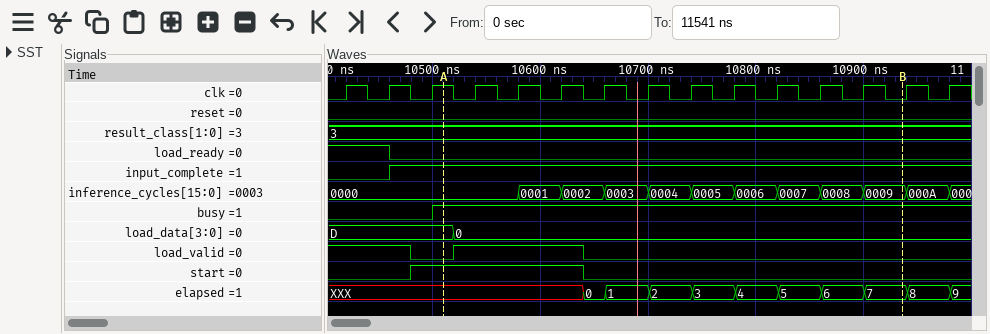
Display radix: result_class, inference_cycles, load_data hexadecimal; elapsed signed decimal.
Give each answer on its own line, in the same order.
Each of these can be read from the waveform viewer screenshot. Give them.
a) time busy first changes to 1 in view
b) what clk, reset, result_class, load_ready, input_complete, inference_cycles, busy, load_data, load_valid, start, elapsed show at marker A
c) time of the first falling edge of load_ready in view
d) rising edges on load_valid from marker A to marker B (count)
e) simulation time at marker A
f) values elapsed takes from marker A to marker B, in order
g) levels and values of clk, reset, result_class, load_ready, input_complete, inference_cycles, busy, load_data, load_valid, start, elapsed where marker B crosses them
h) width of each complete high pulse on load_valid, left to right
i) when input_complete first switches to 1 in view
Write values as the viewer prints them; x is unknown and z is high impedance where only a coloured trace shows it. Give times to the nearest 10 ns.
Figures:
10500 ns
clk=1, reset=0, result_class=3, load_ready=0, input_complete=1, inference_cycles=0000, busy=1, load_data=D, load_valid=0, start=1, elapsed=XXX
10460 ns
1
10510 ns
XXX, 0, 1, 2, 3, 4, 5, 6, 7
clk=0, reset=0, result_class=3, load_ready=0, input_complete=1, inference_cycles=0009, busy=1, load_data=0, load_valid=0, start=0, elapsed=7
120 ns
10460 ns
